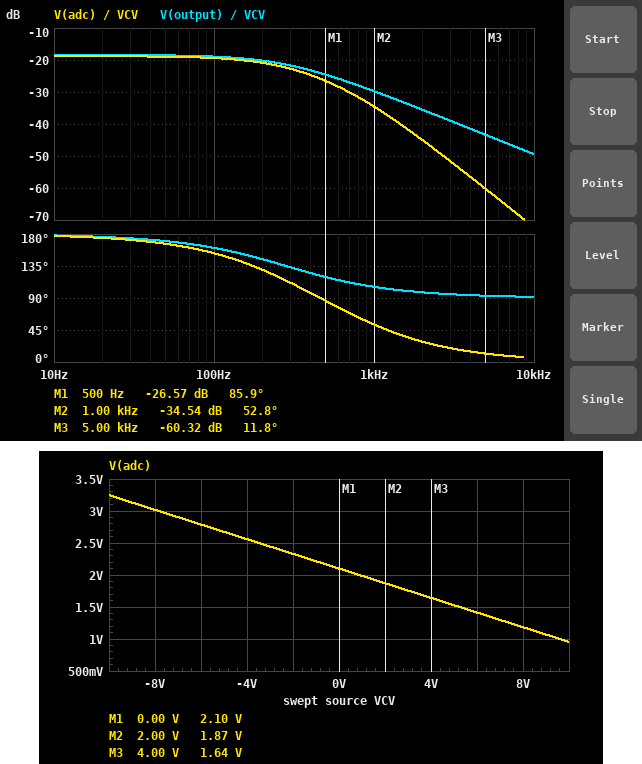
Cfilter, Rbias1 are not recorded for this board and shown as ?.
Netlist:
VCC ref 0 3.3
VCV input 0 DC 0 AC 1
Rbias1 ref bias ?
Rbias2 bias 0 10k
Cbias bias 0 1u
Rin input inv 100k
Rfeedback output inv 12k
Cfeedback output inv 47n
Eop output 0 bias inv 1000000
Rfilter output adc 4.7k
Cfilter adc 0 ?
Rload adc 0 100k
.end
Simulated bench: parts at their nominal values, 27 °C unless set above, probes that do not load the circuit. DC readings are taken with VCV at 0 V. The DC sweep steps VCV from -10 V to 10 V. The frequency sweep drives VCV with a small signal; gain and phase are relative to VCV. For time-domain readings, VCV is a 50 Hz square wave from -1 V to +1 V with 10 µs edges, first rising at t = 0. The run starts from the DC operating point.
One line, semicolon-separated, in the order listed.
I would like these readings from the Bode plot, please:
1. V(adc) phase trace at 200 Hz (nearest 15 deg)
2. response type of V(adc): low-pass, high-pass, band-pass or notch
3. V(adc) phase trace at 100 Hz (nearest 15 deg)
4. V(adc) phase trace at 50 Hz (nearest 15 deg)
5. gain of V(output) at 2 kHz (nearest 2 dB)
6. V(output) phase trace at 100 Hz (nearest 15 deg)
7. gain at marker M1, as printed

135 deg; low-pass; 150 deg; 165 deg; -36 dB; 165 deg; -26.57 dB
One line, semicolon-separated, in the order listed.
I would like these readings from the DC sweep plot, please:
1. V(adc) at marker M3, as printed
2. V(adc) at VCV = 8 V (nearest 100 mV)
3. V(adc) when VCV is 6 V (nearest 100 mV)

1.64 V; 1.2 V; 1.4 V
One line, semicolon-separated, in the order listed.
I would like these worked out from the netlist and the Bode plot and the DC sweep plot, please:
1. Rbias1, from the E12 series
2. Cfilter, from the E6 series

6.8 kΩ; 47 nF
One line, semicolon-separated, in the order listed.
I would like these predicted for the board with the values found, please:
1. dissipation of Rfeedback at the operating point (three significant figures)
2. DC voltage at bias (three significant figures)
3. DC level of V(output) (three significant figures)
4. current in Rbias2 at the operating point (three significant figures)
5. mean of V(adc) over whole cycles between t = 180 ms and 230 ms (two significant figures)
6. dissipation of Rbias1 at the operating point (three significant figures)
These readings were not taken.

4.63 µW; 1.96 V; 2.20 V; 196 µA; 2.1 V; 262 µW
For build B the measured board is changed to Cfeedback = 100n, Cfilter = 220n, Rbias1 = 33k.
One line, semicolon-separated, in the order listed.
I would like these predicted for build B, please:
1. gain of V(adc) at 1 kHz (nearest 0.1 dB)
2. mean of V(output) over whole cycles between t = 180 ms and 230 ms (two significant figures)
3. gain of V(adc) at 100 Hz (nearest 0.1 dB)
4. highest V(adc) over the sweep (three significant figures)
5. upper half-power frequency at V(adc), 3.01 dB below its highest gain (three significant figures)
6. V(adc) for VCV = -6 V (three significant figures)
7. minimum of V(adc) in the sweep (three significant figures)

-52.4 dB; 860 mV; -22.2 dB; 1.97 V; 93.5 Hz; 1.51 V; -325 mV
